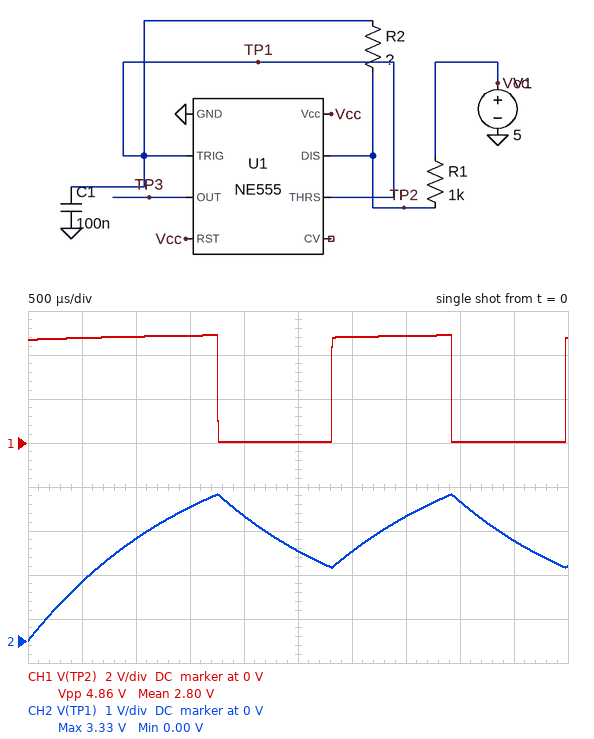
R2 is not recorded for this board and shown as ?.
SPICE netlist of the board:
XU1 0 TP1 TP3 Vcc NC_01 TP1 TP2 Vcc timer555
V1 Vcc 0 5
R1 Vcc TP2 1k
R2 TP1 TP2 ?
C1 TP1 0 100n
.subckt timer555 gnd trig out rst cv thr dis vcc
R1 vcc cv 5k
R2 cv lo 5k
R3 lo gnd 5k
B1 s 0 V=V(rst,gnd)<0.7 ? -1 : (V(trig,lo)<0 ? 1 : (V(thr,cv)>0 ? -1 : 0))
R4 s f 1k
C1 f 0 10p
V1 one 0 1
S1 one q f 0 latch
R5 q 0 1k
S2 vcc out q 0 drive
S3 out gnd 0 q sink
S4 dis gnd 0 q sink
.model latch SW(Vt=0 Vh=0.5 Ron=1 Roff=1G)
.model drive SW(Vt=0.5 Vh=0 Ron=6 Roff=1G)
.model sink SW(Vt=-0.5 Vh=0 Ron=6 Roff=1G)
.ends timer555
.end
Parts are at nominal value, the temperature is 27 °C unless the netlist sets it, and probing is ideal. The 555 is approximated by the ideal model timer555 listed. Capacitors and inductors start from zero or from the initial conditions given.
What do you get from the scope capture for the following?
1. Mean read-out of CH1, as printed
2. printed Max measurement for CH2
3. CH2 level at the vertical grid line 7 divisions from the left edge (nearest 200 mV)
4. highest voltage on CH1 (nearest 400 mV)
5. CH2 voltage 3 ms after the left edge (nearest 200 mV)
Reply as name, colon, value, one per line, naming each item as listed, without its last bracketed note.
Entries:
Mean read-out of CH1, as printed: 2.80 V
printed Max measurement for CH2: 3.33 V
CH2 level at the vertical grid line 7 divisions from the left edge: 2.8 V
highest voltage on CH1: 4.8 V
CH2 voltage 3 ms after the left edge: 2.0 V
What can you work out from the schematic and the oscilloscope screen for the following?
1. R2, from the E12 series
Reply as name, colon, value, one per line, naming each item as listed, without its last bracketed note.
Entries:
R2, from the E12 series: 15 kΩ
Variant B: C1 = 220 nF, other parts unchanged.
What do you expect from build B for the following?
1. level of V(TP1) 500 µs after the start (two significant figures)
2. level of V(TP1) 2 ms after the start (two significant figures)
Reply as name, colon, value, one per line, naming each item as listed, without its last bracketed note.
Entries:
level of V(TP1) 500 µs after the start: 660 mV
level of V(TP1) 2 ms after the start: 2.2 V
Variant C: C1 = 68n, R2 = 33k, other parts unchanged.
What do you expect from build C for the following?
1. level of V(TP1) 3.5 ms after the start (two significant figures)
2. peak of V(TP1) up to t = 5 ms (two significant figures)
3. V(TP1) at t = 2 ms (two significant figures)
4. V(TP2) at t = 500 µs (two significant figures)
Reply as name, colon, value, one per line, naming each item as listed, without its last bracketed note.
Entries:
level of V(TP1) 3.5 ms after the start: 2.2 V
peak of V(TP1) up to t = 5 ms: 3.3 V
V(TP1) at t = 2 ms: 2.9 V
V(TP2) at t = 500 µs: 4.9 V
